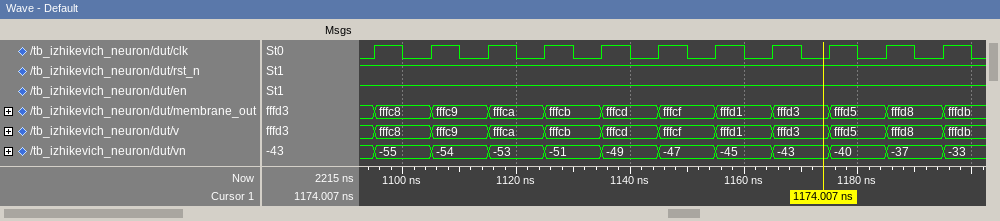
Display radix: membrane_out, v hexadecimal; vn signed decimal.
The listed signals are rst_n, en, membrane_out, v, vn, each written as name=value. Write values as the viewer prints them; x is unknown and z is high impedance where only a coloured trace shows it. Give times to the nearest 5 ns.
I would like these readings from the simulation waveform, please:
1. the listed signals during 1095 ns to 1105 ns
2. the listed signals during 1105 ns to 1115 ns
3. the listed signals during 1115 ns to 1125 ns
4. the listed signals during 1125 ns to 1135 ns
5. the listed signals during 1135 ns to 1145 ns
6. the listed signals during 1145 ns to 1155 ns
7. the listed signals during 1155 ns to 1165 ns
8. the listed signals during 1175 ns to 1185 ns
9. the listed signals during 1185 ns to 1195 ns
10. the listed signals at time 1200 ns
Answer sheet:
rst_n=1, en=1, membrane_out=fffc8, v=fffc8, vn=-55
rst_n=1, en=1, membrane_out=fffc9, v=fffc9, vn=-54
rst_n=1, en=1, membrane_out=fffca, v=fffca, vn=-53
rst_n=1, en=1, membrane_out=fffcb, v=fffcb, vn=-51
rst_n=1, en=1, membrane_out=fffcd, v=fffcd, vn=-49
rst_n=1, en=1, membrane_out=fffcf, v=fffcf, vn=-47
rst_n=1, en=1, membrane_out=fffd1, v=fffd1, vn=-45
rst_n=1, en=1, membrane_out=fffd5, v=fffd5, vn=-40
rst_n=1, en=1, membrane_out=fffd8, v=fffd8, vn=-37
rst_n=1, en=1, membrane_out=fffdb, v=fffdb, vn=-33
